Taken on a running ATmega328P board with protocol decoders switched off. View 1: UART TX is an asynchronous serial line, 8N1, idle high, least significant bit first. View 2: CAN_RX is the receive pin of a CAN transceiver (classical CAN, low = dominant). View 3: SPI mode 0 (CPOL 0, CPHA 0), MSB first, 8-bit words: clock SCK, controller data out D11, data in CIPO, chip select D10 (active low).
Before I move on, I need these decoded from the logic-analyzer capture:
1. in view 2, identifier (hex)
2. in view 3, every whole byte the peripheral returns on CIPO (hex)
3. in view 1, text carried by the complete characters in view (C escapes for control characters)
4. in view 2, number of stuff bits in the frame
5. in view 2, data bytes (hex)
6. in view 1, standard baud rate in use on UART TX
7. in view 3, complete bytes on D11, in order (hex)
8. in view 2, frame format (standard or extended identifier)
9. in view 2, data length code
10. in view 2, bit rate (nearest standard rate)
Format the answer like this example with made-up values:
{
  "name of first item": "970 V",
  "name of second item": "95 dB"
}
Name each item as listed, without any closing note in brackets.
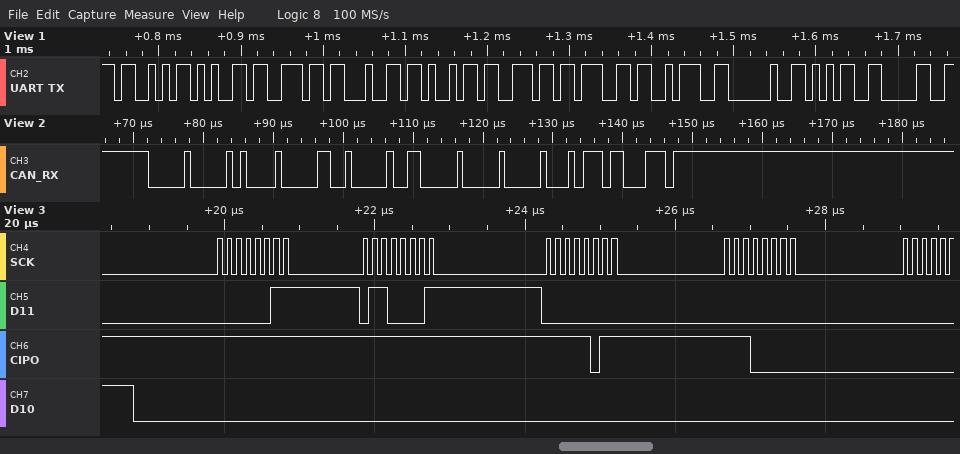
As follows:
{
  "in view 2, identifier": "0x001",
  "in view 3, every whole byte the peripheral returns on CIPO": "0xFF 0xFF 0xFB 0xE0",
  "in view 1, text carried by the complete characters in view": "\"Sending: 50\"",
  "in view 2, number of stuff bits in the frame": "7",
  "in view 2, data bytes": "12 03 00 00",
  "in view 1, standard baud rate in use on UART TX": "115200 baud",
  "in view 3, complete bytes on D11, in order": "0x03 0x61 0x00 0x00",
  "in view 2, frame format": "standard",
  "in view 2, data length code": "4",
  "in view 2, bit rate": "1000 kbit/s"
}
